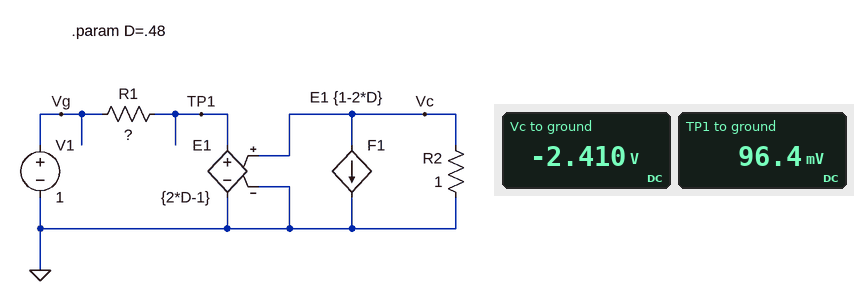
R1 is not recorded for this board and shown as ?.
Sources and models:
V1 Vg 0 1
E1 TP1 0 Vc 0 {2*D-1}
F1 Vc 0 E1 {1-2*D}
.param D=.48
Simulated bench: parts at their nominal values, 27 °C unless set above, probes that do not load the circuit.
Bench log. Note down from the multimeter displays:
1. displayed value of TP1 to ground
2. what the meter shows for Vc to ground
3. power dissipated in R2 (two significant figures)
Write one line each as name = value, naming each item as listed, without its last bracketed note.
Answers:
displayed value of TP1 to ground = 96.4 mV
what the meter shows for Vc to ground = -2.410 V
power dissipated in R2 = 5.8 W
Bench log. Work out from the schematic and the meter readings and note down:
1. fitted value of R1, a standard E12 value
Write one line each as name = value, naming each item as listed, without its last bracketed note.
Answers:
fitted value of R1, a standard E12 value = 0.015 Ω
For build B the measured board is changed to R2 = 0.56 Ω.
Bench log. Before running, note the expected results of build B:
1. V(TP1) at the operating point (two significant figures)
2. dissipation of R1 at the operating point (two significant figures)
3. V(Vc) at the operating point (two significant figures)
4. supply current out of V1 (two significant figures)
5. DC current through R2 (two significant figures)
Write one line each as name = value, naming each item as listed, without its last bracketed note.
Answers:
V(TP1) at the operating point = 56 mV
dissipation of R1 at the operating point = 59 W
V(Vc) at the operating point = -1.4 V
supply current out of V1 = 63 A
DC current through R2 = 2.5 A
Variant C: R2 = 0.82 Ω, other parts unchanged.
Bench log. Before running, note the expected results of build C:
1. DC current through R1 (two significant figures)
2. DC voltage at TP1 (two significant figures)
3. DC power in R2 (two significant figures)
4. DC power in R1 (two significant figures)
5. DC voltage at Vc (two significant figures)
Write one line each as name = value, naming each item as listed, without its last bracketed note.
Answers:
DC current through R1 = 61 A
DC voltage at TP1 = 80 mV
DC power in R2 = 4.9 W
DC power in R1 = 56 W
DC voltage at Vc = -2.0 V
